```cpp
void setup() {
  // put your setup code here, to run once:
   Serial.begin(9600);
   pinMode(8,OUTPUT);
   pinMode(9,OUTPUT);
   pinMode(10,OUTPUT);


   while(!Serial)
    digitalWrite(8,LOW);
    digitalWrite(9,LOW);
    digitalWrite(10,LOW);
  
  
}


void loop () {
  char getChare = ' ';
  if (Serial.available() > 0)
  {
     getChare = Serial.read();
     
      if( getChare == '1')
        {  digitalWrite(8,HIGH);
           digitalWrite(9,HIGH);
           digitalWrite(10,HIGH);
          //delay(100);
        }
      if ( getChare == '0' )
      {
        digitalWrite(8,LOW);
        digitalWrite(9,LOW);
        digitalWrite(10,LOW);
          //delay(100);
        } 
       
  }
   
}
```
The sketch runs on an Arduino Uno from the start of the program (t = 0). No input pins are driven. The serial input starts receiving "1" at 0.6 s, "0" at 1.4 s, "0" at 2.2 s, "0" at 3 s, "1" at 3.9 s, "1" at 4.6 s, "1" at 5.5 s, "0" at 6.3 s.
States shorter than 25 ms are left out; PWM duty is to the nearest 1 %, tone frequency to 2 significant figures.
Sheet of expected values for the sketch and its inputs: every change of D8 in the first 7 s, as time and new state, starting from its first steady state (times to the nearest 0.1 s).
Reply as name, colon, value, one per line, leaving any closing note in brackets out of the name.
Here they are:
every change of D8 in the first 7 s, as time and new state, starting from its first steady state: 0 s low; 0.6 s high; 1.4 s low; 3.9 s high; 6.3 s low
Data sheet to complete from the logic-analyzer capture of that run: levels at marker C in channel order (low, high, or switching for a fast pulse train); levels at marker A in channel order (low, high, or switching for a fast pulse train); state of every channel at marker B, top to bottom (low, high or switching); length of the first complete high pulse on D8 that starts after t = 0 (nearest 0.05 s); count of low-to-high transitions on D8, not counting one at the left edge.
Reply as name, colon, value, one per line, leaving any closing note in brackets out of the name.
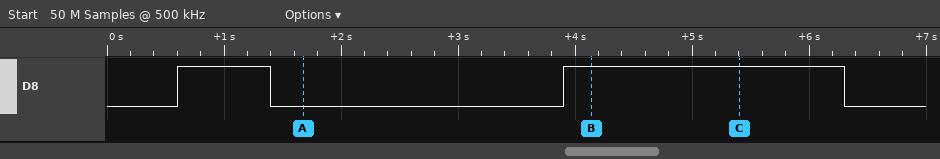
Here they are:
levels at marker C in channel order: D8 high
levels at marker A in channel order: D8 low
state of every channel at marker B, top to bottom: D8 high
length of the first complete high pulse on D8 that starts after t = 0: 0.80 s
count of low-to-high transitions on D8, not counting one at the left edge: 2
